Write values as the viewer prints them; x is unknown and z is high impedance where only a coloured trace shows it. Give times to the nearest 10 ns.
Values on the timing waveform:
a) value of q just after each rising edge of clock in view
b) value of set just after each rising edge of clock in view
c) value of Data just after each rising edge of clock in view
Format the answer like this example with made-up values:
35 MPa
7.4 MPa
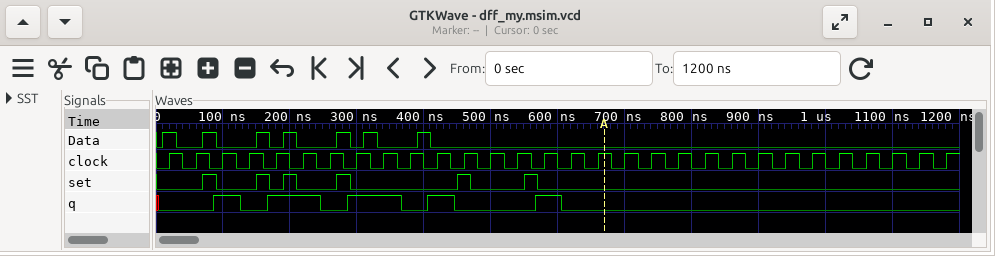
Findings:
0 0 1 0 1 1 0 1 1 0 1 0 0 0 1 0 0 0 0 0 0 0 0 0 0 0 0 0 0 0
0 0 0 0 0 0 0 0 0 0 0 1 0 0 0 0 0 0 0 0 0 0 0 0 0 0 0 0 0 0
1 0 0 0 0 0 0 0 0 0 0 0 0 0 0 0 0 0 0 0 0 0 0 0 0 0 0 0 0 0
